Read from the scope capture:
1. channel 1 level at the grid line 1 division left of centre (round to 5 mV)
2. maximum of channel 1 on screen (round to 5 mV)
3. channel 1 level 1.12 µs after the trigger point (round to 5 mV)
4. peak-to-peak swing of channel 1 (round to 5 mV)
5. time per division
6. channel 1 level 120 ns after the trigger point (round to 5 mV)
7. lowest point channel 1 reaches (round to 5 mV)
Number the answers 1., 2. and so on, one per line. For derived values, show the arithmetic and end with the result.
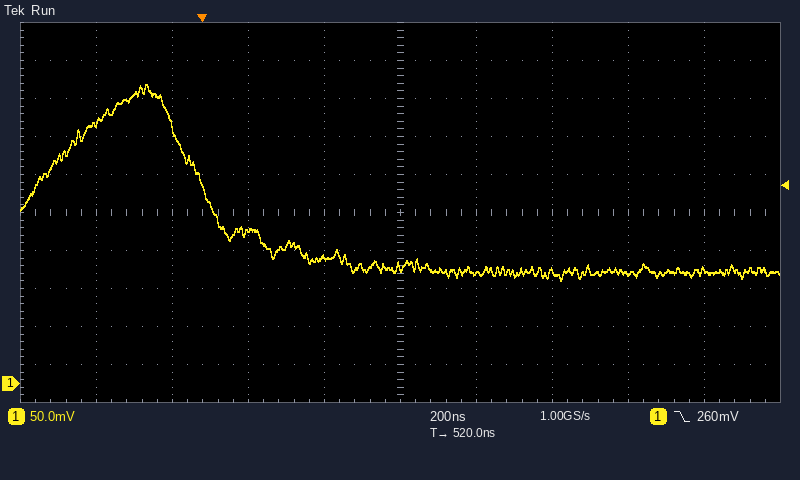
1. 165 mV
2. 395 mV
3. 145 mV
4. 395 mV − (135 mV) = 260 mV
5. 200 ns
6. 200 mV
7. 135 mV
